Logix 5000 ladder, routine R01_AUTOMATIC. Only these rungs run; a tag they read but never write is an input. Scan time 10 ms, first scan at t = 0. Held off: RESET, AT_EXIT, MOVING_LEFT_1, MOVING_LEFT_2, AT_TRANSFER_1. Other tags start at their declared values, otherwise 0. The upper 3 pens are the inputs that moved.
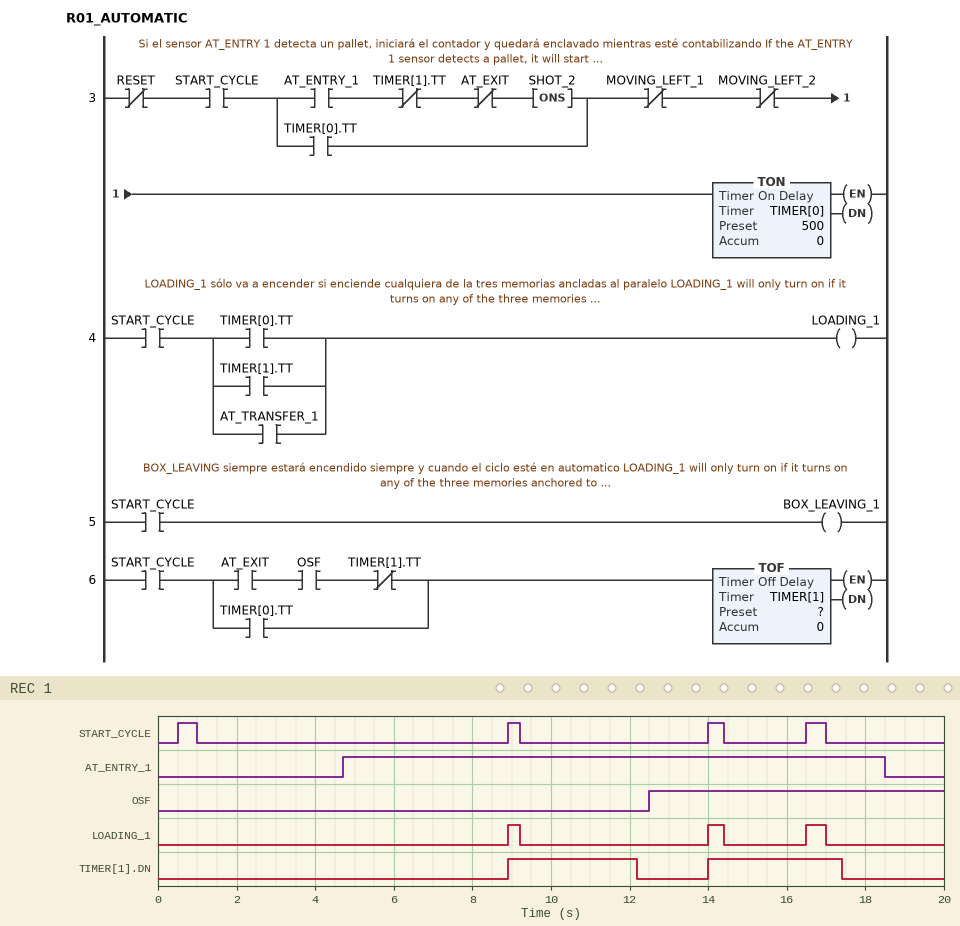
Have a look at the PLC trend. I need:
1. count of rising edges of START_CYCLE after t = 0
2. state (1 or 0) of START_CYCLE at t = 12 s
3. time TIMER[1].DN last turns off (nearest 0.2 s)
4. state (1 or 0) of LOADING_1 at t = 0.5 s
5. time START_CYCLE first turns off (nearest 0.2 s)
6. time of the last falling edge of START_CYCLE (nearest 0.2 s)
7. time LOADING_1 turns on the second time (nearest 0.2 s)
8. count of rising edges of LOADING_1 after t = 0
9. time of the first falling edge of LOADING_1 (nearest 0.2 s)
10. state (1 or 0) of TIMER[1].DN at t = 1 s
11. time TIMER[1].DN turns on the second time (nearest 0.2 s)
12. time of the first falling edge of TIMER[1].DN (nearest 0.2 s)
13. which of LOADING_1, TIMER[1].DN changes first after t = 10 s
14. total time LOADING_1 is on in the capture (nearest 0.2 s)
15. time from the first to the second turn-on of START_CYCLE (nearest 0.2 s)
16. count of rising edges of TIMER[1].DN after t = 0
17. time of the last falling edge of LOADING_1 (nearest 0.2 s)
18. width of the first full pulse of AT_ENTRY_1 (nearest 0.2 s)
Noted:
4
0
17.4 s
0
1.0 s
17.0 s
14.0 s
3
9.2 s
0
14.0 s
12.2 s
TIMER[1].DN
1.2 s
8.4 s
2
17.0 s
13.8 s
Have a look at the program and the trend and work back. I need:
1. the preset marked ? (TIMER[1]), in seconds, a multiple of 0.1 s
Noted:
3.0 s
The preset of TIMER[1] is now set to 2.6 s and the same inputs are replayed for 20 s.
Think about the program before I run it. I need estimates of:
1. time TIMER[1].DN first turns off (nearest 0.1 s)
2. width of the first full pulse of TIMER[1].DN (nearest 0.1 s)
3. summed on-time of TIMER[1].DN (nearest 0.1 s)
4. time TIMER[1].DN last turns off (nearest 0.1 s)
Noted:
11.8 s
2.9 s
5.9 s
17.0 s
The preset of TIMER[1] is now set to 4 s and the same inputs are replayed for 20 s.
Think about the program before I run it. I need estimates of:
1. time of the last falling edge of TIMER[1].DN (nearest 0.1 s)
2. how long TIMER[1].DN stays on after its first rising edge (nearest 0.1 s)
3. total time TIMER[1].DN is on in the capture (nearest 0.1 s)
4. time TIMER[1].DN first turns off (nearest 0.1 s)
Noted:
18.4 s
4.3 s
8.7 s
13.2 s
